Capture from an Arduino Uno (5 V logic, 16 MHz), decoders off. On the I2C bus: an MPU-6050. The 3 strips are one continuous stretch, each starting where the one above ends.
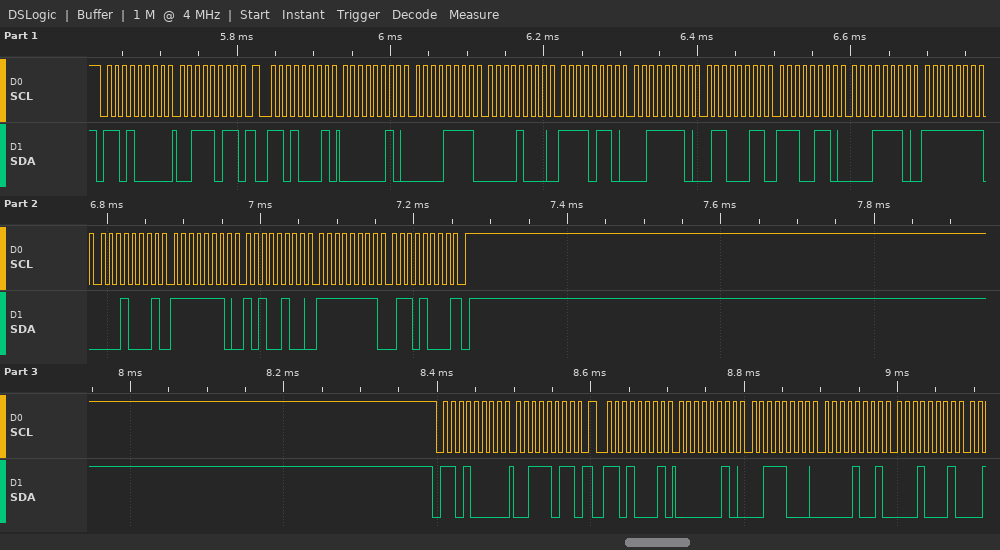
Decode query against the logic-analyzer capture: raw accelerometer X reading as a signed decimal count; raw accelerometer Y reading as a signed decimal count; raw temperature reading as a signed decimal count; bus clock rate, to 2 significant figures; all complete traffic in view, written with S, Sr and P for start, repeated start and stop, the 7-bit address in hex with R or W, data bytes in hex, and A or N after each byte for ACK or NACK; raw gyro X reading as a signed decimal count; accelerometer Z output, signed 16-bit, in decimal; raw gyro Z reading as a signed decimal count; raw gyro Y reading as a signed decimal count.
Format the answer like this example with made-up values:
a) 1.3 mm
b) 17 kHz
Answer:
a) 527
b) 2294
c) -6626
d) 100 kHz
e) S 68W A 3B A Sr 68R A 02 A 0F A 08 A F6 A 3E A 63 A E6 A 1E A FF A 11 A FE A A4 A FF A 68 N P S 68W A 3B A Sr 68R A 02 A 38 A 09 A 11 A
f) -239
g) 15971
h) -152
i) -348
